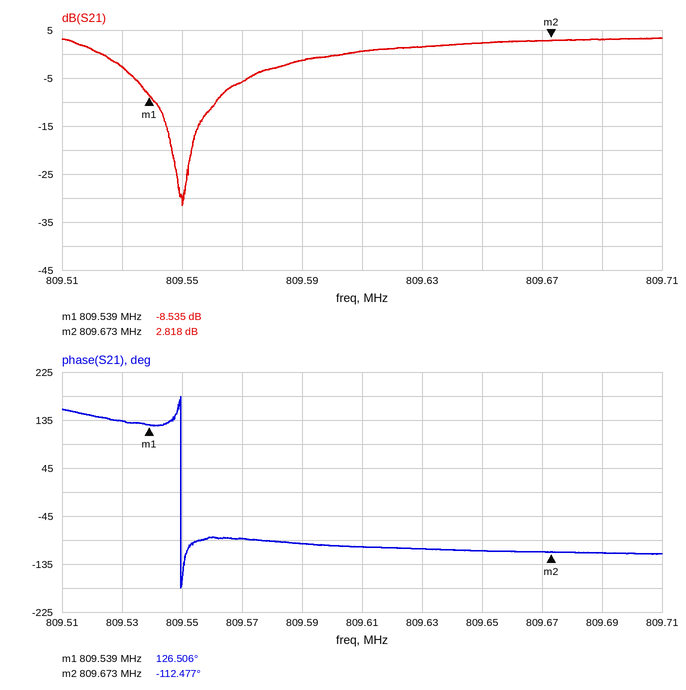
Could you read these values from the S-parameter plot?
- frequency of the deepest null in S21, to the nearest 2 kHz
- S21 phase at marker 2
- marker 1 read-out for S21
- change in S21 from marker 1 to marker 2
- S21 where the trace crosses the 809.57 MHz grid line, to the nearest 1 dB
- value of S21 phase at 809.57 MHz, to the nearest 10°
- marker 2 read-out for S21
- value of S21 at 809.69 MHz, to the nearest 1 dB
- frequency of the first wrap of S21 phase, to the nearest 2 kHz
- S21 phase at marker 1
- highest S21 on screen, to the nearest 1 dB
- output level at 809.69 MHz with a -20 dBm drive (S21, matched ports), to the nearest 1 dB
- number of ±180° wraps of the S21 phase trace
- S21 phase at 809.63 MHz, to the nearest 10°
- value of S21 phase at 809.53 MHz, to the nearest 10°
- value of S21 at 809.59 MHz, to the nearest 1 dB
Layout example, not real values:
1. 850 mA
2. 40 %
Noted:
1. 809.550 MHz
2. -112.477°
3. -8.535 dB
4. 11.353 dB
5. -6 dB
6. -90°
7. 2.818 dB
8. 3 dB
9. 809.550 MHz
10. 126.506°
11. 3 dB
12. -17 dBm
13. 1
14. -110°
15. 130°
16. -1 dB
